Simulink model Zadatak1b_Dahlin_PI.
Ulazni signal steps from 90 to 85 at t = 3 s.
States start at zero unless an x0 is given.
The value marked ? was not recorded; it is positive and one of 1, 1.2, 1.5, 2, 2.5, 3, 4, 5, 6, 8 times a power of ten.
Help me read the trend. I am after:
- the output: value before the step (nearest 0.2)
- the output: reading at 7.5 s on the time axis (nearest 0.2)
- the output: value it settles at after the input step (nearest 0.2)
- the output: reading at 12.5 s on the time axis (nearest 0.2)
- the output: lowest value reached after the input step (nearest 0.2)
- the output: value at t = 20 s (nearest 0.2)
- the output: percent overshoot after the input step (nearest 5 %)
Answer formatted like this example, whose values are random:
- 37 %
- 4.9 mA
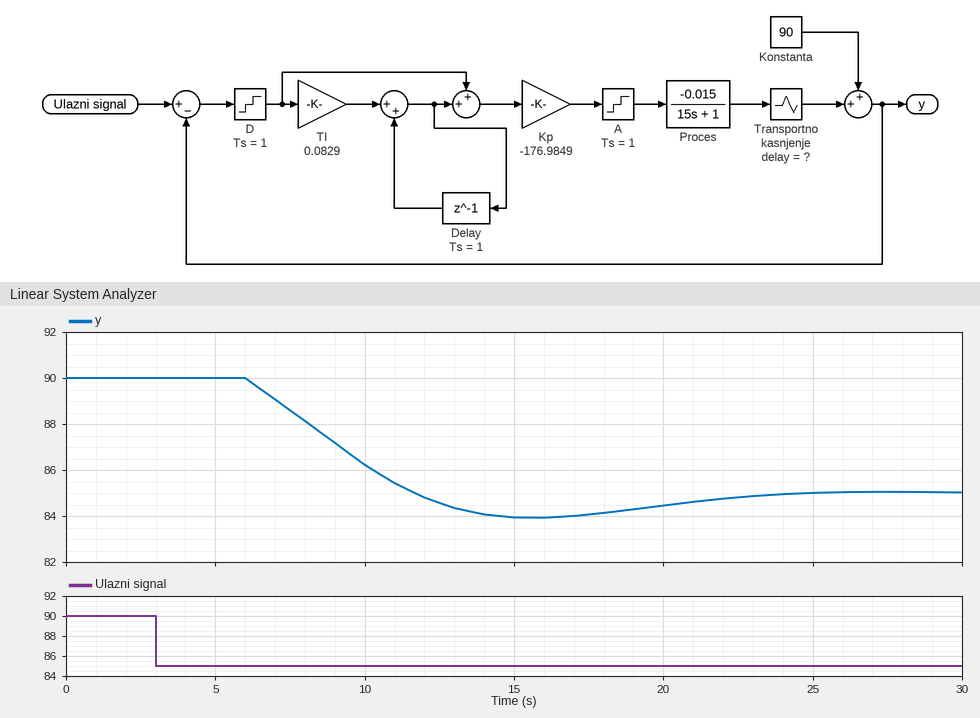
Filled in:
- 90.0
- 88.6
- 85.0
- 84.6
- 84.0
- 84.4
- 20 %
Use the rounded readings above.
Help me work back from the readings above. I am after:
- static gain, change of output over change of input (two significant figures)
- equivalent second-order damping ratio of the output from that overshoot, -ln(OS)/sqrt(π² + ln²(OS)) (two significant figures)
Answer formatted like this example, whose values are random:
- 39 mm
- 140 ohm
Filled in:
- 1.0
- 0.46
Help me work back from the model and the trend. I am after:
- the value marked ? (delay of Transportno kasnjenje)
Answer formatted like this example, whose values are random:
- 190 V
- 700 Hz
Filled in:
- 3
